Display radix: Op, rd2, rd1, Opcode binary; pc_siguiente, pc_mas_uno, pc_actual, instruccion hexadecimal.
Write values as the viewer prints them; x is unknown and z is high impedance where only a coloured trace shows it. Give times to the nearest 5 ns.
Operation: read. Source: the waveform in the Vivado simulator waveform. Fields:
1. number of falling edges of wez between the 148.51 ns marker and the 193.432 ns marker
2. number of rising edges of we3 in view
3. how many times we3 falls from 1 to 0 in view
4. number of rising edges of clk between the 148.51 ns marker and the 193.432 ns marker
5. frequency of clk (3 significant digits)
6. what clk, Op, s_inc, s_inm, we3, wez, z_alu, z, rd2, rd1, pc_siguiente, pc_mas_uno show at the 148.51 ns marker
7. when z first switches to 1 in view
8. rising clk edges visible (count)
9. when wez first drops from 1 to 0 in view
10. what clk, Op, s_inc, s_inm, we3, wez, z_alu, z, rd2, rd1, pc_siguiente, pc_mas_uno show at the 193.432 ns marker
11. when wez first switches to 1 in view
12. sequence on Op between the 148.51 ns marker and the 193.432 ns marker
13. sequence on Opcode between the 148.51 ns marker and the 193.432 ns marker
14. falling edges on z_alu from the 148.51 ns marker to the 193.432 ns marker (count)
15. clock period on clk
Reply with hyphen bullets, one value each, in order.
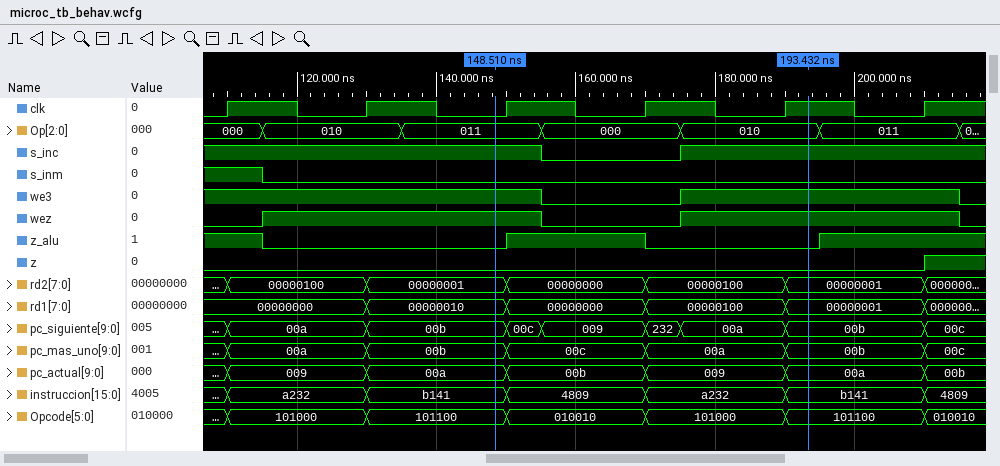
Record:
- 1
- 1
- 2
- 3
- 50.0 MHz
- clk=0, Op=011, s_inc=1, s_inm=0, we3=1, wez=1, z_alu=0, z=0, rd2=00000001, rd1=00000010, pc_siguiente=00b, pc_mas_uno=00b
- 210 ns
- 6
- 155 ns
- clk=1, Op=010, s_inc=1, s_inm=0, we3=1, wez=1, z_alu=0, z=0, rd2=00000001, rd1=00000001, pc_siguiente=00b, pc_mas_uno=00b
- 115 ns
- 011, 000, 010
- 101100, 010010, 101000, 101100
- 1
- 20 ns
